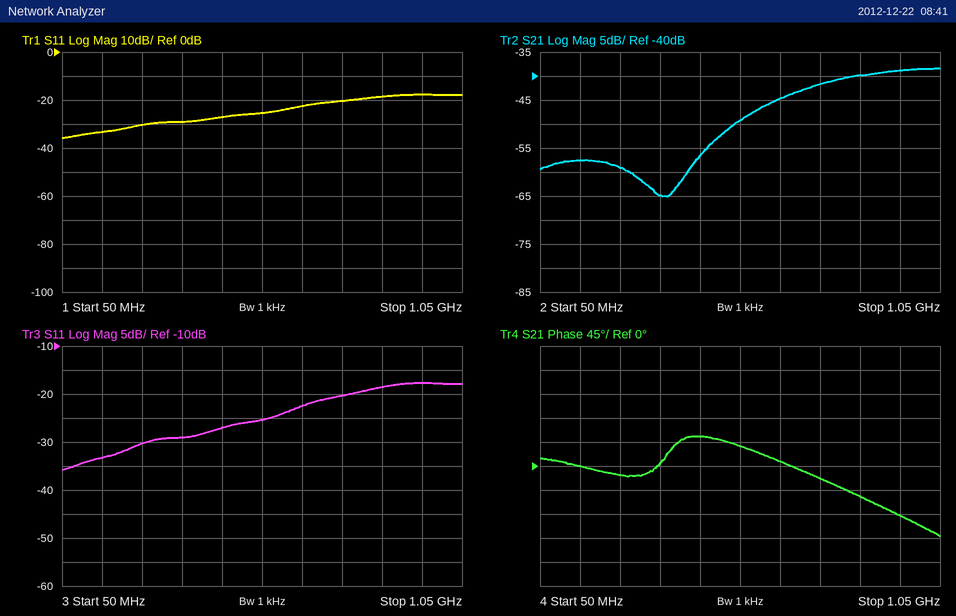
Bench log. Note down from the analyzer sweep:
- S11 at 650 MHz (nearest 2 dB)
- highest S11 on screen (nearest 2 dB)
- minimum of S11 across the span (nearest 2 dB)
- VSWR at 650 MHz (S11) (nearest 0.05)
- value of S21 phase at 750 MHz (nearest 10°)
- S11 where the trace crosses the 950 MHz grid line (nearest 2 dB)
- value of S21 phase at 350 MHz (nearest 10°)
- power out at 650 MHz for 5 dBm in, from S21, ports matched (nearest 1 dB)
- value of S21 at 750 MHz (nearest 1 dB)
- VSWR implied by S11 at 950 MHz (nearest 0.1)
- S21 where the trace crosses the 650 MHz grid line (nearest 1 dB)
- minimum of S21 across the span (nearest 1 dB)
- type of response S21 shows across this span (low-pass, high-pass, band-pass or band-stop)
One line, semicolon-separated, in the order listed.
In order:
-22 dB; -18 dB; -36 dB; 1.15; -20°; -18 dB; 0°; -40 dBm; -42 dB; 1.3; -45 dB; -65 dB; high-pass
